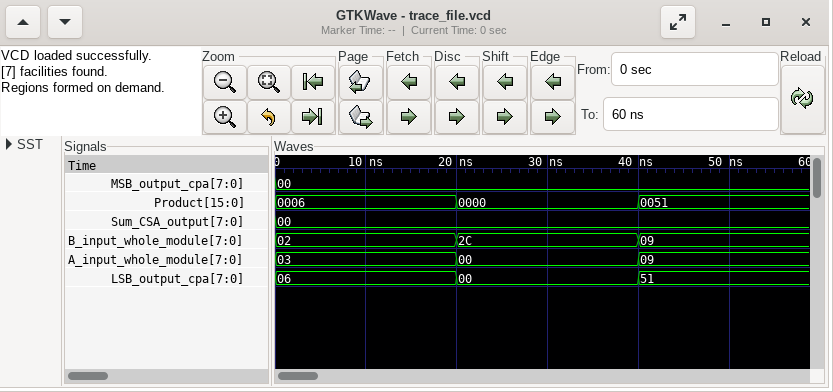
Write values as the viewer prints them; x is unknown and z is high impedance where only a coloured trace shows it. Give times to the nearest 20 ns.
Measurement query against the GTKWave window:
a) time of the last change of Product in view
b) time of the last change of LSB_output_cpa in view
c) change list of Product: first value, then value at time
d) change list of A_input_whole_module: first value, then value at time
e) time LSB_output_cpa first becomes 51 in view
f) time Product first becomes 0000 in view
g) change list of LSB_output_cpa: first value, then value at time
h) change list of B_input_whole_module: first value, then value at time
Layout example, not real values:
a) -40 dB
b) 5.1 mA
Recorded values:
a) 40 ns
b) 40 ns
c) 0006, 0000 at 20 ns, 0051 at 40 ns
d) 03, 00 at 20 ns, 09 at 40 ns
e) 40 ns
f) 20 ns
g) 06, 00 at 20 ns, 51 at 40 ns
h) 02, 2C at 20 ns, 09 at 40 ns
